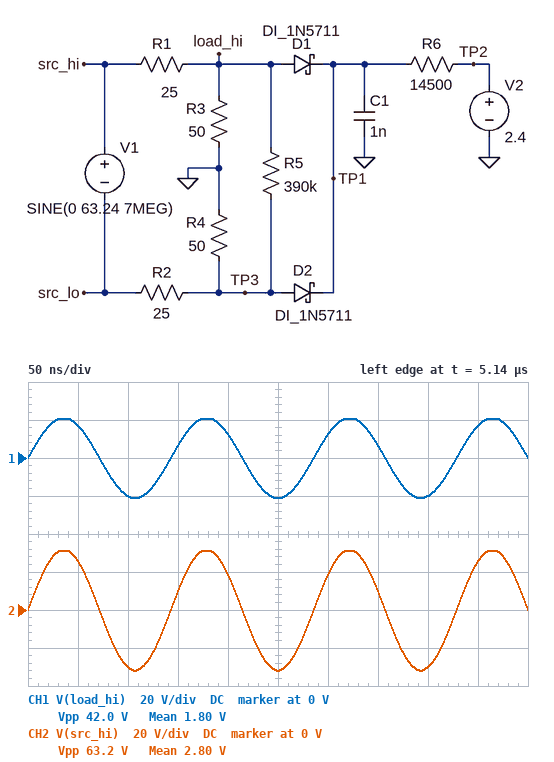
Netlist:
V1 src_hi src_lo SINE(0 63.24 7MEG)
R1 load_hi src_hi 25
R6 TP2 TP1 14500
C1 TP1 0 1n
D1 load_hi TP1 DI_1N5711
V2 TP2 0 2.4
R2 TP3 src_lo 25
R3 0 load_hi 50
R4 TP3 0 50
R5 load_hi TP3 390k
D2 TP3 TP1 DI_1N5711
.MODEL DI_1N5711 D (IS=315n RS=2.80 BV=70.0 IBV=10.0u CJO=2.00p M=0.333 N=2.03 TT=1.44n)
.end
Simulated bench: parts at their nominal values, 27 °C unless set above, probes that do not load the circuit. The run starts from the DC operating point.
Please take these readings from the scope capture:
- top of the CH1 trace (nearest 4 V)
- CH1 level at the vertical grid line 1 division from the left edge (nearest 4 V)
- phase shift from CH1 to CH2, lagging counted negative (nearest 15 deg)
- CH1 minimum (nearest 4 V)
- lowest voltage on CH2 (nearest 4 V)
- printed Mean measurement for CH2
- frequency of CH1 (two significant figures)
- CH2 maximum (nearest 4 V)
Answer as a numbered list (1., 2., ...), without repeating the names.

1. 20 V
2. 16 V
3. 0 deg
4. -20 V
5. -32 V
6. 2.80 V
7. 7.0 MHz
8. 32 V
